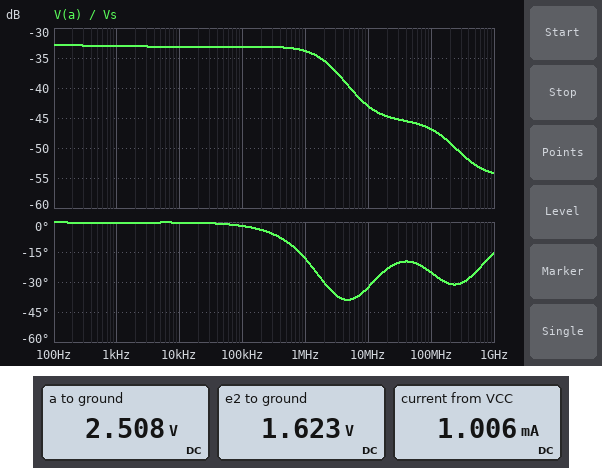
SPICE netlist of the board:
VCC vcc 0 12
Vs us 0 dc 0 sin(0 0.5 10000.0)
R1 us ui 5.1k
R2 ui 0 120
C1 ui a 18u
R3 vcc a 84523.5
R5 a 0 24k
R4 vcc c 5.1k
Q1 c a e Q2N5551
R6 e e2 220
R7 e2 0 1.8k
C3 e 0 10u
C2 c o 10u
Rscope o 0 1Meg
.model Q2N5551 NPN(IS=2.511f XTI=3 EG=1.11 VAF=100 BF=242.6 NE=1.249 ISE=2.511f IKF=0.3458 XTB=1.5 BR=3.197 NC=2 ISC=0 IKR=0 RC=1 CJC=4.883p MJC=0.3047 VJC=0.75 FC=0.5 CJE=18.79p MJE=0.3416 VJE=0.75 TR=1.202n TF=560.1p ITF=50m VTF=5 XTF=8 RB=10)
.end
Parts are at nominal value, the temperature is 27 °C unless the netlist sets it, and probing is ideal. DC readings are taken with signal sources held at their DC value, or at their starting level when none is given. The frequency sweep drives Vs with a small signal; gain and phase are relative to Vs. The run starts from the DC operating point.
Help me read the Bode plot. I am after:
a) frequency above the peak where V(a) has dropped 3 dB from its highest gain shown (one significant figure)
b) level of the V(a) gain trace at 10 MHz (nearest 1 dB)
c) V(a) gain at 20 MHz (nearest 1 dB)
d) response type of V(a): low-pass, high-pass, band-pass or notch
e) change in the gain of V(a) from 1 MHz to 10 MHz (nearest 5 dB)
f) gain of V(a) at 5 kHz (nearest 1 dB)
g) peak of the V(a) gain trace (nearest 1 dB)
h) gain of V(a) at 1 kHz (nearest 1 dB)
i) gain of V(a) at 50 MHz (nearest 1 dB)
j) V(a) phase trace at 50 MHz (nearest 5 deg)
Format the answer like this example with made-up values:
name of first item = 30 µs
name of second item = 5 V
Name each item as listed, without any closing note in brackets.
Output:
frequency above the peak where V(a) has dropped 3 dB from its highest gain shown = 2 MHz
level of the V(a) gain trace at 10 MHz = -43 dB
V(a) gain at 20 MHz = -45 dB
response type of V(a): low-pass, high-pass, band-pass or notch = low-pass
change in the gain of V(a) from 1 MHz to 10 MHz = -10 dB
gain of V(a) at 5 kHz = -33 dB
peak of the V(a) gain trace = -33 dB
gain of V(a) at 1 kHz = -33 dB
gain of V(a) at 50 MHz = -46 dB
V(a) phase trace at 50 MHz = -20 deg
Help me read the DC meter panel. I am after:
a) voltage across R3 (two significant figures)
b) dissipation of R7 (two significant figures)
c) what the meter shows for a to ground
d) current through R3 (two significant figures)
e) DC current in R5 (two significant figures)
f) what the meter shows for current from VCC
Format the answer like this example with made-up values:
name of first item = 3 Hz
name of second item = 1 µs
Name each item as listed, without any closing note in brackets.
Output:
voltage across R3 = 9.5 V
dissipation of R7 = 1.5 mW
what the meter shows for a to ground = 2.508 V
current through R3 = 110 µA
DC current in R5 = 100 µA
what the meter shows for current from VCC = 1.006 mA
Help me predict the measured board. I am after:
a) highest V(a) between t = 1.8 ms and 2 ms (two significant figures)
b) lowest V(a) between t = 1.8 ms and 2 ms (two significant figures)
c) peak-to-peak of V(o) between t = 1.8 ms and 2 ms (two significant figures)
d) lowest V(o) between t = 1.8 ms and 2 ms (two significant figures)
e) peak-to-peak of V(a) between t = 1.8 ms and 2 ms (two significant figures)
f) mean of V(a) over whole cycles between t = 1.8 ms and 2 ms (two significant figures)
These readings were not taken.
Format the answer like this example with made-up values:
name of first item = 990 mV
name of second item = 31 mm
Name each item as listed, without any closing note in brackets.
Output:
highest V(a) between t = 1.8 ms and 2 ms = 2.5 V
lowest V(a) between t = 1.8 ms and 2 ms = 2.5 V
peak-to-peak of V(o) between t = 1.8 ms and 2 ms = 3.6 V
lowest V(o) between t = 1.8 ms and 2 ms = -2.0 V
peak-to-peak of V(a) between t = 1.8 ms and 2 ms = 22 mV
mean of V(a) over whole cycles between t = 1.8 ms and 2 ms = 2.5 V
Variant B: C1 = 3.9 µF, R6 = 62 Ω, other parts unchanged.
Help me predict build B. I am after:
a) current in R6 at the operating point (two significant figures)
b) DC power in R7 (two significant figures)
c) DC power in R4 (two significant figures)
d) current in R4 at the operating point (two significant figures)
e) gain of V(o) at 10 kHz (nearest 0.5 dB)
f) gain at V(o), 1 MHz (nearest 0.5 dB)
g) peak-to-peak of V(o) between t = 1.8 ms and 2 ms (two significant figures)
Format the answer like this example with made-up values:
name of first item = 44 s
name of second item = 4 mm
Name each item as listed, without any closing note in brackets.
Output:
current in R6 at the operating point = 970 µA
DC power in R7 = 1.7 mW
DC power in R4 = 4.7 mW
current in R4 at the operating point = 960 µA
gain of V(o) at 10 kHz = 12.0 dB
gain at V(o), 1 MHz = 11.0 dB
peak-to-peak of V(o) between t = 1.8 ms and 2 ms = 3.9 V
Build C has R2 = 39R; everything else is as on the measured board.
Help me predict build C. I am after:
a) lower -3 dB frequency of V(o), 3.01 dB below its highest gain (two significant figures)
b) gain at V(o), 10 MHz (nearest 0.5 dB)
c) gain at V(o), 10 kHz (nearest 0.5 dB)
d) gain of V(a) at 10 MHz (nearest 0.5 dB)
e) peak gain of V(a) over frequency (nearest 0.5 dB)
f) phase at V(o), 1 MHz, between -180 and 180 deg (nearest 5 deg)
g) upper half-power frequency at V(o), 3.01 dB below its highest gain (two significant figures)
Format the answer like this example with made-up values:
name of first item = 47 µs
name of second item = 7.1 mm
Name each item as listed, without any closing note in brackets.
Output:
lower -3 dB frequency of V(o), 3.01 dB below its highest gain = 530 Hz
gain at V(o), 10 MHz = -6.0 dB
gain at V(o), 10 kHz = 2.0 dB
gain of V(a) at 10 MHz = -47.0 dB
peak gain of V(a) over frequency = -42.5 dB
phase at V(o), 1 MHz, between -180 and 180 deg = 165 deg
upper half-power frequency at V(o), 3.01 dB below its highest gain = 4.5 MHz
